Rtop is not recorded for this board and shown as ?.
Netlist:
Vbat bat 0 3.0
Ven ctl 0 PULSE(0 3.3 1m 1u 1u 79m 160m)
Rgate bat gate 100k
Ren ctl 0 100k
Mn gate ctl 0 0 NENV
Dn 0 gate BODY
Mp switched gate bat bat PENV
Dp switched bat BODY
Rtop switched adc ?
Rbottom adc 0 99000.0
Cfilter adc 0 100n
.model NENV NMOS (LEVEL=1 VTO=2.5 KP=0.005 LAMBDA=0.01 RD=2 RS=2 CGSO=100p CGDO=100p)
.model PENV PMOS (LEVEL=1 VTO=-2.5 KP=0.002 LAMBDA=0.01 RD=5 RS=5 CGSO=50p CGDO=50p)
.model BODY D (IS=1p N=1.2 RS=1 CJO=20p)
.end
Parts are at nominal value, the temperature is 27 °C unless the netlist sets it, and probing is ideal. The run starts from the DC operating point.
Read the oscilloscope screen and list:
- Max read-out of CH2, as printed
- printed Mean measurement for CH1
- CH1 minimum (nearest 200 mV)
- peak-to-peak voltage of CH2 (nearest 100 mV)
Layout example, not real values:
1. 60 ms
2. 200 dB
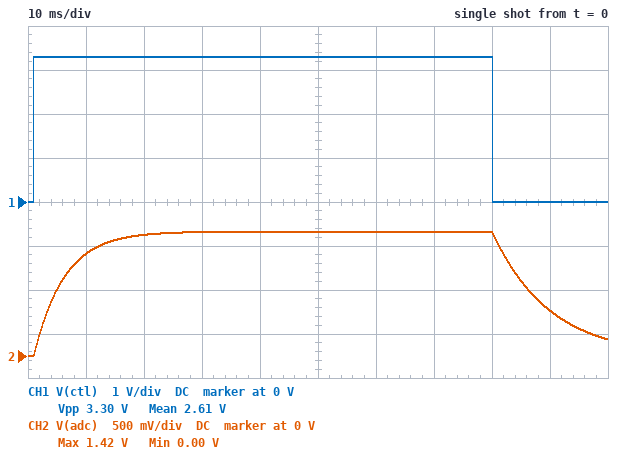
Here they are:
1. 1.42 V
2. 2.61 V
3. 0 V
4. 1.4 V
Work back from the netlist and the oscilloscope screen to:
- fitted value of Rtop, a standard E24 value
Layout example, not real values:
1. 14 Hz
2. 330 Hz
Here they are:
1. 110 kΩ
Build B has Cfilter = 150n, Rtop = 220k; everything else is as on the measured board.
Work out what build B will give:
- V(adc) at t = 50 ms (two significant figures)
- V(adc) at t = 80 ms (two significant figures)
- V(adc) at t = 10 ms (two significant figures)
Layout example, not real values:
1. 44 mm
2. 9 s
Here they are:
1. 920 mV
2. 930 mV
3. 540 mV
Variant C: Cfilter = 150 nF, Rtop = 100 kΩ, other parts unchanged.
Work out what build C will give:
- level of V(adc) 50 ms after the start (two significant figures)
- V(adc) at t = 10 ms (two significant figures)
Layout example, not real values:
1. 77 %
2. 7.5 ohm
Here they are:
1. 1.5 V
2. 1.0 V
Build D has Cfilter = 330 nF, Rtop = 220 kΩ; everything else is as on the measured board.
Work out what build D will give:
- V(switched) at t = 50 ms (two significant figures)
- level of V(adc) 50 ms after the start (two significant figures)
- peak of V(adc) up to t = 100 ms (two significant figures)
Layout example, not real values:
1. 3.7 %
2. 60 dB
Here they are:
1. 3.0 V
2. 820 mV
3. 900 mV
